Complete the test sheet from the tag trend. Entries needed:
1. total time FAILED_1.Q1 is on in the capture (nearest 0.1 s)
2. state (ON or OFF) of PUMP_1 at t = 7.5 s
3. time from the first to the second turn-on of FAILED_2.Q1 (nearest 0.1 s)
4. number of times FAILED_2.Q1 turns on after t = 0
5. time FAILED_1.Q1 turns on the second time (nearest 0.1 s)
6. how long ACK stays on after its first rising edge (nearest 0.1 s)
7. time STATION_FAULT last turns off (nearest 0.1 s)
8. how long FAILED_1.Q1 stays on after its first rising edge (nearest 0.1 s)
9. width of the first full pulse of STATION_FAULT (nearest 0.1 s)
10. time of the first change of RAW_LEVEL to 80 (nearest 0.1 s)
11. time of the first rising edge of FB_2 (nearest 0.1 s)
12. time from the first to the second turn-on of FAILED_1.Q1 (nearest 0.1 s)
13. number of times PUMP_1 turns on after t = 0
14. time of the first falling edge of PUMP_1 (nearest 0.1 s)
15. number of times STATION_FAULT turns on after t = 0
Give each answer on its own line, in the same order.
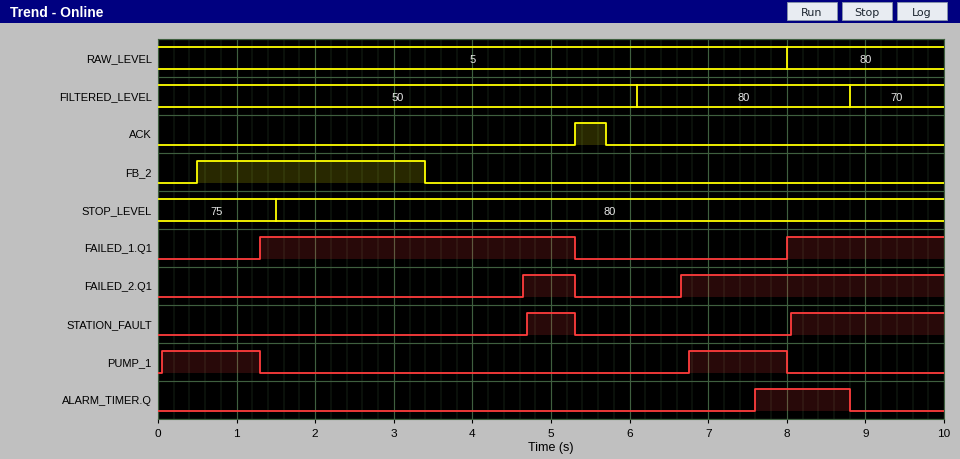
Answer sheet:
6.0 s
ON
2.0 s
2
8.0 s
0.4 s
5.3 s
4.0 s
0.6 s
8.0 s
0.5 s
6.7 s
2
1.3 s
2
